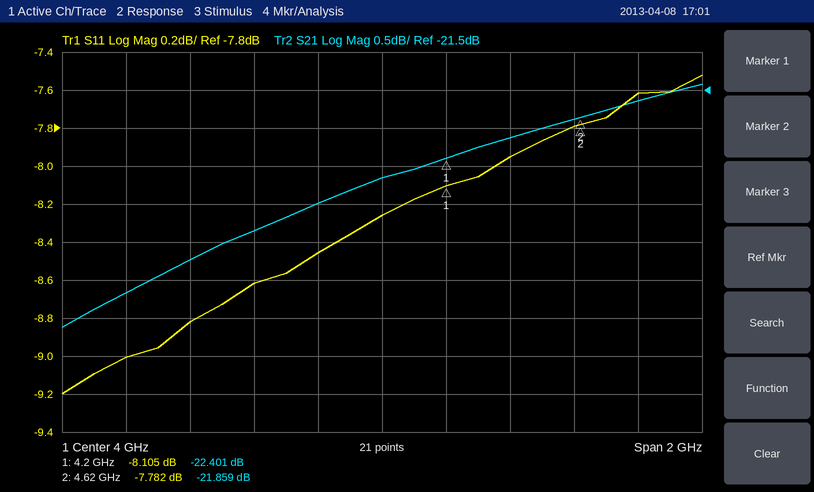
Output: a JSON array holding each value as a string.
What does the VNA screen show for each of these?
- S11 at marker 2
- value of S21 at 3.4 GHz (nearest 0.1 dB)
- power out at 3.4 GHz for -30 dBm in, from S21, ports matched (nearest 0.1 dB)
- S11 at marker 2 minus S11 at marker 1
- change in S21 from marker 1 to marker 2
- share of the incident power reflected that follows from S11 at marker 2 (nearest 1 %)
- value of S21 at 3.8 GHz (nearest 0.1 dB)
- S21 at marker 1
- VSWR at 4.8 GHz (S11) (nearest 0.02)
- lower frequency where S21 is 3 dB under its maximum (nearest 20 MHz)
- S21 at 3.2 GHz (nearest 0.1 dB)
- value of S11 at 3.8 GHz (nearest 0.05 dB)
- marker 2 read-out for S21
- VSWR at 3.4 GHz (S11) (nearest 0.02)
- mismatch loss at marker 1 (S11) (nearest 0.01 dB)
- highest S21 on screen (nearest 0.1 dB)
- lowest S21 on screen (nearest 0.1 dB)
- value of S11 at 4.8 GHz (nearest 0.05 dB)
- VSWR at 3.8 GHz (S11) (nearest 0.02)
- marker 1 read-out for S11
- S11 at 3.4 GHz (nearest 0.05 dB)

["-7.782 dB", "-23.7 dB", "-53.7 dBm", "0.323 dB", "0.542 dB", "17 %", "-23.0 dB", "-22.401 dB", "2.42", "3.08 GHz", "-24.2 dB", "-8.45 dB", "-21.859 dB", "2.14", "0.73 dB", "-21.4 dB", "-24.6 dB", "-7.60 dB", "2.22", "-8.105 dB", "-8.80 dB"]
